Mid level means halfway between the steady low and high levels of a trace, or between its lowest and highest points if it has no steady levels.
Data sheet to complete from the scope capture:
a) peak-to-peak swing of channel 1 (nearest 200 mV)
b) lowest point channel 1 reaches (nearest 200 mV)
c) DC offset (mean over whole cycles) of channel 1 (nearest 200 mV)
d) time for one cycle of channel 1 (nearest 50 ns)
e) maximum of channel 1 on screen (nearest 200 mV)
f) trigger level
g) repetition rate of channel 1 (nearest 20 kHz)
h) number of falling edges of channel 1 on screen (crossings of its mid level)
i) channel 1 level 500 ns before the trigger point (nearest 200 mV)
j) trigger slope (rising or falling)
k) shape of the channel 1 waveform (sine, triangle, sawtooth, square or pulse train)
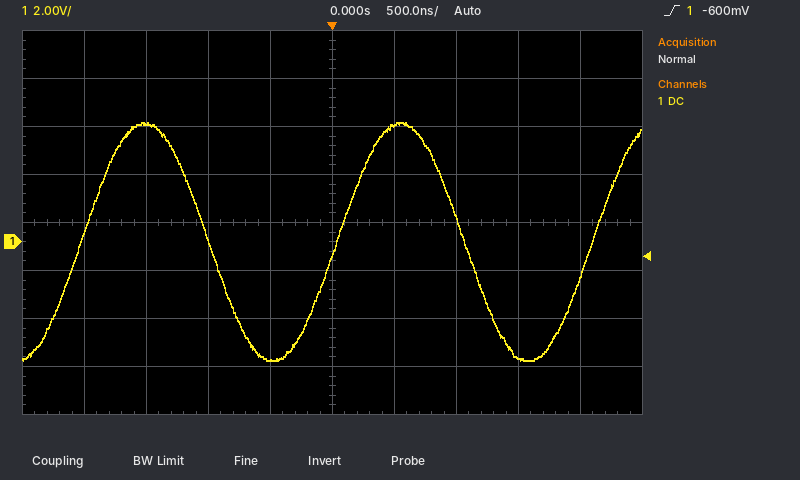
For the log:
10.0 V
-5.0 V
0.0 V
2.05 µs
5.0 V
-600 mV
480 kHz
2
-5.0 V
rising
sine
